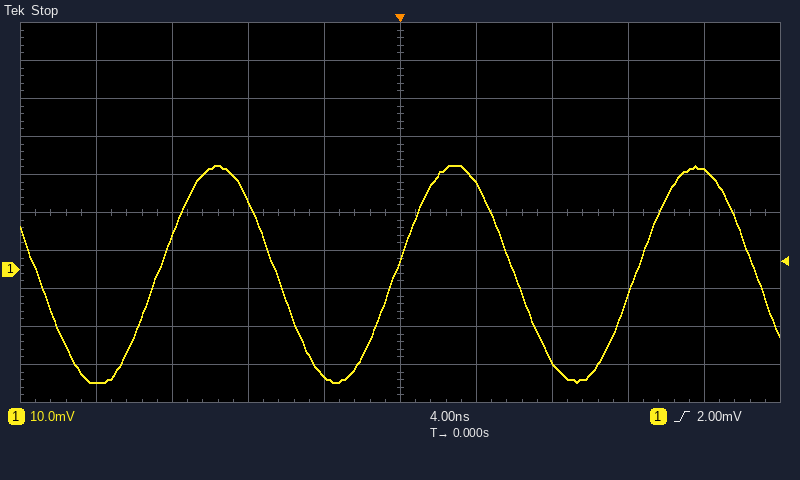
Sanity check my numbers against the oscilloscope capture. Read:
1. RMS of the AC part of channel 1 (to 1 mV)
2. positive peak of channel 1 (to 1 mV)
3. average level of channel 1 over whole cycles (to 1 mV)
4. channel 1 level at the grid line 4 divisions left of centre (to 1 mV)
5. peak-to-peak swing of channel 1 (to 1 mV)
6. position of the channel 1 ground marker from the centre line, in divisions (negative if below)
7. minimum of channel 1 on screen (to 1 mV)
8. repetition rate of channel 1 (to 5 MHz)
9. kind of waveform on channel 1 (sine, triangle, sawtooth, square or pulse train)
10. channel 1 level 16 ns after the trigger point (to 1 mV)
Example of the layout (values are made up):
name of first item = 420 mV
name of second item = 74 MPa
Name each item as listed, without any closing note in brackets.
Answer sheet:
RMS of the AC part of channel 1 = 20 mV
positive peak of channel 1 = 27 mV
average level of channel 1 over whole cycles = -1 mV
channel 1 level at the grid line 4 divisions left of centre = -30 mV
peak-to-peak swing of channel 1 = 57 mV
position of the channel 1 ground marker from the centre line, in divisions = -1.5 div
minimum of channel 1 on screen = -30 mV
repetition rate of channel 1 = 80 MHz
kind of waveform on channel 1 = sine
channel 1 level 16 ns after the trigger point = 26 mV
